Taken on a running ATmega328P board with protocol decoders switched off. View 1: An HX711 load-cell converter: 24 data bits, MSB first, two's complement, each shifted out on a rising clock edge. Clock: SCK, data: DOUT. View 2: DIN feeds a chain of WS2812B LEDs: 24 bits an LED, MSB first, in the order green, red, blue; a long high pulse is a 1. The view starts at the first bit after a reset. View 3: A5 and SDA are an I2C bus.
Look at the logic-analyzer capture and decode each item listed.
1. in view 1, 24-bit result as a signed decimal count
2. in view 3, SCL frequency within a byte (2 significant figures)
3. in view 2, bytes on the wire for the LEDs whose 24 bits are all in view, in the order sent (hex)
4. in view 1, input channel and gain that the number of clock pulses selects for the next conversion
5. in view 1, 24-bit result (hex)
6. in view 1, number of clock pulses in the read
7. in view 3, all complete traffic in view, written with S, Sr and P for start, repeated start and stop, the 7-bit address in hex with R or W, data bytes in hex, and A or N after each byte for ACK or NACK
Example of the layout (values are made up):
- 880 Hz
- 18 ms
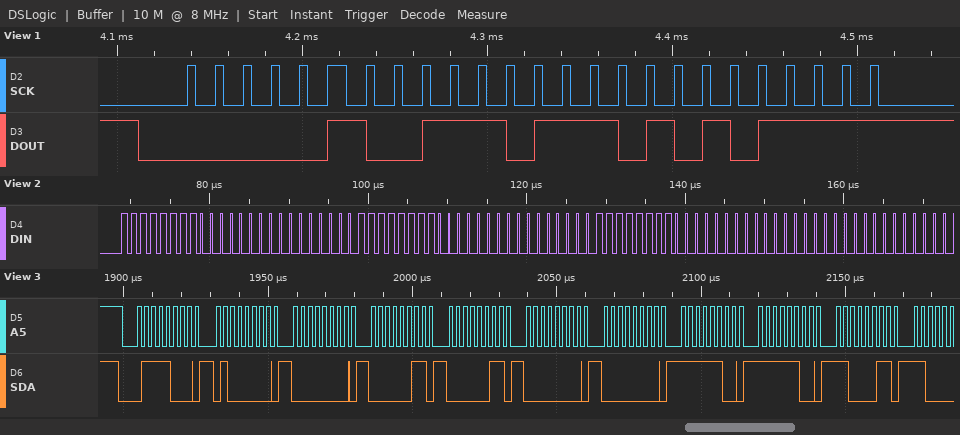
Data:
- 323247
- 400 kHz
- FF 00 00 FF 00 00 FF 00 00
- channel A, gain 128
- 0x04EEAF
- 25
- S 3CW A 40 A 00 A 03 A 03 A 00 A 00 A FC A FC A C3 A
